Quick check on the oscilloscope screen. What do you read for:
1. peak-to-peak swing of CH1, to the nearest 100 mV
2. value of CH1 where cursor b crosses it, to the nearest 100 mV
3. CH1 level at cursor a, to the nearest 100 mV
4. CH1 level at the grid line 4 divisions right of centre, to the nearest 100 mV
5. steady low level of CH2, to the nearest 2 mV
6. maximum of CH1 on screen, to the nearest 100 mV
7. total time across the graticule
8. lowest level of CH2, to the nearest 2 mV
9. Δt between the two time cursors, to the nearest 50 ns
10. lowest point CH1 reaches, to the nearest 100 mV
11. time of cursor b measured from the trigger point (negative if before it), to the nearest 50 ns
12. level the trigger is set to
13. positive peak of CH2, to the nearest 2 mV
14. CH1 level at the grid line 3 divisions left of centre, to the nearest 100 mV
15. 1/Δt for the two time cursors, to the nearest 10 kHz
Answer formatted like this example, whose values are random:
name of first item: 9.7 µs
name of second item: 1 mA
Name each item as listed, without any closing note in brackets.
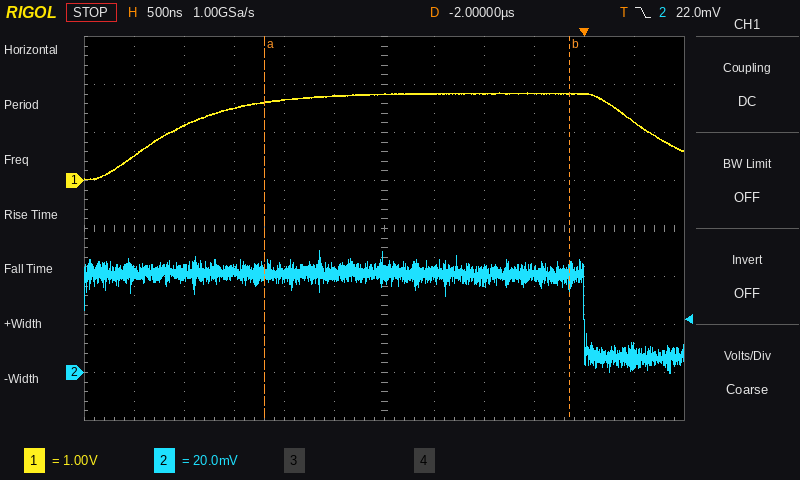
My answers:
peak-to-peak swing of CH1, to the nearest 100 mV: 1.8 V
value of CH1 where cursor b crosses it, to the nearest 100 mV: 1.8 V
CH1 level at cursor a, to the nearest 100 mV: 1.6 V
CH1 level at the grid line 4 divisions right of centre, to the nearest 100 mV: 1.8 V
steady low level of CH2, to the nearest 2 mV: 6 mV
maximum of CH1 on screen, to the nearest 100 mV: 1.8 V
total time across the graticule: 6 µs
lowest level of CH2, to the nearest 2 mV: 0 mV
Δt between the two time cursors, to the nearest 50 ns: 3.05 µs
lowest point CH1 reaches, to the nearest 100 mV: 0.0 V
time of cursor b measured from the trigger point (negative if before it), to the nearest 50 ns: -150 ns
level the trigger is set to: 22.0 mV
positive peak of CH2, to the nearest 2 mV: 50 mV
CH1 level at the grid line 3 divisions left of centre, to the nearest 100 mV: 1.5 V
1/Δt for the two time cursors, to the nearest 10 kHz: 330 kHz
